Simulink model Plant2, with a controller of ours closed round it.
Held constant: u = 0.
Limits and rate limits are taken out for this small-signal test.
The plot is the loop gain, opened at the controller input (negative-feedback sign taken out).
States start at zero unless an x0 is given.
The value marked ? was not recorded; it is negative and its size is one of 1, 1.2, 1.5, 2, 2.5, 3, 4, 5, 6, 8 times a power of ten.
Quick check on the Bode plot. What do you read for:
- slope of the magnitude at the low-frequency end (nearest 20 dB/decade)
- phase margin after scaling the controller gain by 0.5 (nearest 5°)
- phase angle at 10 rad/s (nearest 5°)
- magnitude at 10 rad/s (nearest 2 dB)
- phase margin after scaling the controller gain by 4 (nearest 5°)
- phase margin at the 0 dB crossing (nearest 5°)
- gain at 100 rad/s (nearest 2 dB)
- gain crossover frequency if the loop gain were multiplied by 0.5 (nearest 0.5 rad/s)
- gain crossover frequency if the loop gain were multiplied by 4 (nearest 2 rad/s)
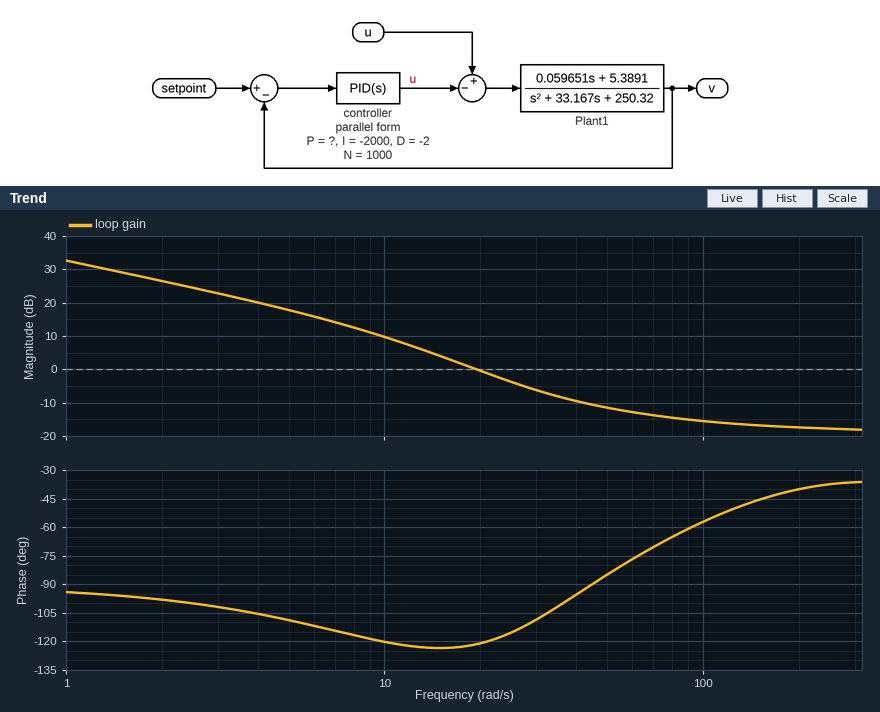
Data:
-20 dB/decade
55°
-120°
10 dB
100°
60°
-16 dB
13.0 rad/s
54 rad/s
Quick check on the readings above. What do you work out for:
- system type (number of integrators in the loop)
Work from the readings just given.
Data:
1
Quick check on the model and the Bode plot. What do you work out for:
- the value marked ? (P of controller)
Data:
-100
